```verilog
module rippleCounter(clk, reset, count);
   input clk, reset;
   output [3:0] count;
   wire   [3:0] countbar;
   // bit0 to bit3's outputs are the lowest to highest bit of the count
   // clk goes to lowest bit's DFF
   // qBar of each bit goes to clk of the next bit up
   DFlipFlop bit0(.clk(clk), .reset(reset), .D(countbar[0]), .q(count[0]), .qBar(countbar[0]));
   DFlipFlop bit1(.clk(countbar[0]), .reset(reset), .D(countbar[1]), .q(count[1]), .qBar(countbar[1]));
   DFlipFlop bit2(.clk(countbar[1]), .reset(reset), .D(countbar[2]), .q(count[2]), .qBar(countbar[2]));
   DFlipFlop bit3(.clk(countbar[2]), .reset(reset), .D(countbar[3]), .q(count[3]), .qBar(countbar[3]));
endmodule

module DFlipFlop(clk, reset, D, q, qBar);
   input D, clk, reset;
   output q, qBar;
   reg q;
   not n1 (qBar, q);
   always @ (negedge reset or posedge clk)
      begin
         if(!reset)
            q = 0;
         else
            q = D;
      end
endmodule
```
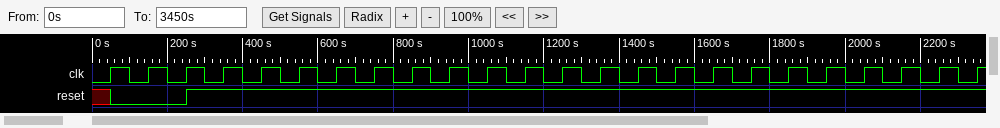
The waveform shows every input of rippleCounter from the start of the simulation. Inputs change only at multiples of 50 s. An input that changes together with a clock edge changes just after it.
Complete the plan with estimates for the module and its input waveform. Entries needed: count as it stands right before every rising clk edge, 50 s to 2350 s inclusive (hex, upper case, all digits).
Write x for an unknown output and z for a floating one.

x, 0, 0, 0, 1, 2, 3, 4, 5, 6, 7, 8, 9, A, B, C, D, E, F, 0, 1, 2, 3, 4
